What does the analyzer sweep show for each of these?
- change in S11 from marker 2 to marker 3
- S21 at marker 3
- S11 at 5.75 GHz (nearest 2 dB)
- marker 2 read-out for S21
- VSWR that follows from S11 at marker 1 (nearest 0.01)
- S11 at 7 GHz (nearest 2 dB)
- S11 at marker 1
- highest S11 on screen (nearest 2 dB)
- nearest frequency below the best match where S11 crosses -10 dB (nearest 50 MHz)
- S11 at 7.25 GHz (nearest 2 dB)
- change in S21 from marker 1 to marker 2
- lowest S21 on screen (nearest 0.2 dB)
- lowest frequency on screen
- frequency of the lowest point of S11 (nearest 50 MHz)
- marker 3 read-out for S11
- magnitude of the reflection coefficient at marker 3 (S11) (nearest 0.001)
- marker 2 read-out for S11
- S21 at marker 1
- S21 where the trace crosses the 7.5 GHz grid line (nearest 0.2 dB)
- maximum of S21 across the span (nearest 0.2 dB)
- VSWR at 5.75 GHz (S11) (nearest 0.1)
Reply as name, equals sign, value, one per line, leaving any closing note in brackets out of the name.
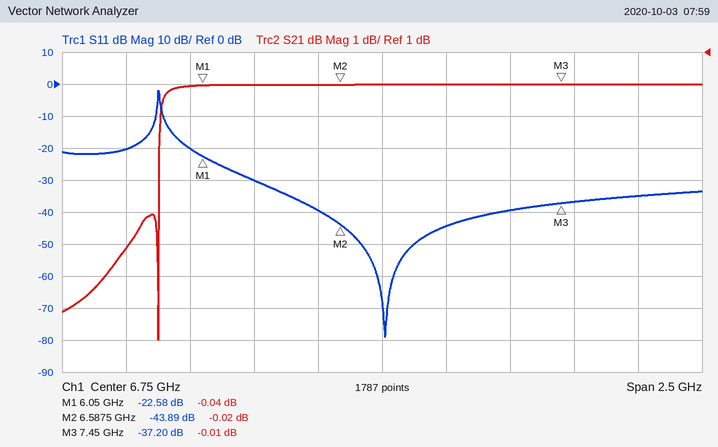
change in S11 from marker 2 to marker 3 = 6.69 dB
S21 at marker 3 = -0.01 dB
S11 at 5.75 GHz = -20 dB
marker 2 read-out for S21 = -0.02 dB
VSWR that follows from S11 at marker 1 = 1.16
S11 at 7 GHz = -44 dB
S11 at marker 1 = -22.58 dB
highest S11 on screen = -2 dB
nearest frequency below the best match where S11 crosses -10 dB = 5.90 GHz
S11 at 7.25 GHz = -40 dB
change in S21 from marker 1 to marker 2 = 0.02 dB
lowest S21 on screen = -8.0 dB
lowest frequency on screen = 5.5 GHz
frequency of the lowest point of S11 = 6.75 GHz
marker 3 read-out for S11 = -37.20 dB
magnitude of the reflection coefficient at marker 3 (S11) = 0.014
marker 2 read-out for S11 = -43.89 dB
S21 at marker 1 = -0.04 dB
S21 where the trace crosses the 7.5 GHz grid line = 0.0 dB
maximum of S21 across the span = 0.0 dB
VSWR at 5.75 GHz (S11) = 1.2
